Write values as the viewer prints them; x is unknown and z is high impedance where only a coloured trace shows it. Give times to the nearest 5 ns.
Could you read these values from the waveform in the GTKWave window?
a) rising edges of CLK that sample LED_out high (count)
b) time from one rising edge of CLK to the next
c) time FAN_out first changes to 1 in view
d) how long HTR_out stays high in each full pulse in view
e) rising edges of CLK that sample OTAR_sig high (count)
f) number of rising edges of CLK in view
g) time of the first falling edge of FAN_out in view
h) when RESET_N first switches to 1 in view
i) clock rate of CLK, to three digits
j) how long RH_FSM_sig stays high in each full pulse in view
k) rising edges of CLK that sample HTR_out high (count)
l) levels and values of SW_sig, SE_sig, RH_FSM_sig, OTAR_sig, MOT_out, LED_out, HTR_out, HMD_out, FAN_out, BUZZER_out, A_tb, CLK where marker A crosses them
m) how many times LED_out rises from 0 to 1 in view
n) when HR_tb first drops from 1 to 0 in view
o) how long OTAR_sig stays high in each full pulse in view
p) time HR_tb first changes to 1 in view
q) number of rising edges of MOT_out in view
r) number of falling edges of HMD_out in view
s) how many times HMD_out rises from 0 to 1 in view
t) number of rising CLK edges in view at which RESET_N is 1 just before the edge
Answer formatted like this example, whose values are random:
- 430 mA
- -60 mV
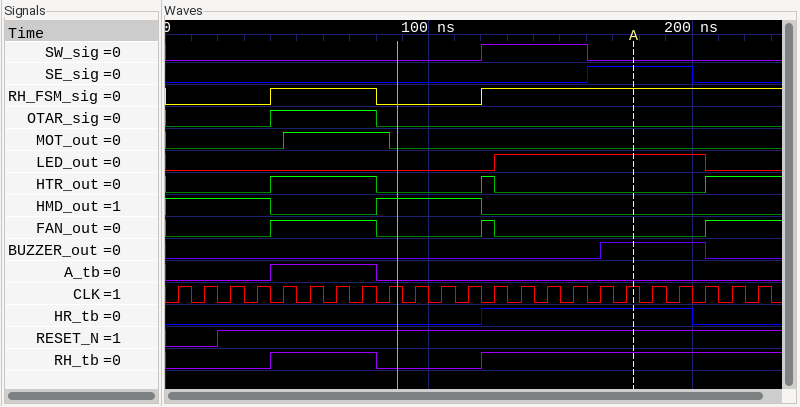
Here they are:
- 8
- 10 ns
- 40 ns
- 40 ns, 5 ns
- 4
- 23
- 80 ns
- 20 ns
- 100 MHz
- 40 ns
- 7
- SW_sig=0, SE_sig=1, RH_FSM_sig=1, OTAR_sig=0, MOT_out=0, LED_out=1, HTR_out=0, HMD_out=0, FAN_out=0, BUZZER_out=1, A_tb=0, CLK=1
- 1
- 200 ns
- 40 ns
- 120 ns
- 1
- 2
- 1
- 21
